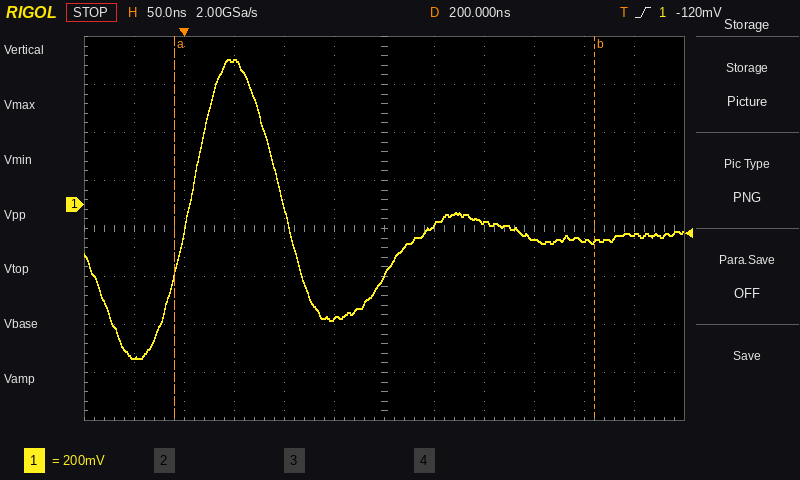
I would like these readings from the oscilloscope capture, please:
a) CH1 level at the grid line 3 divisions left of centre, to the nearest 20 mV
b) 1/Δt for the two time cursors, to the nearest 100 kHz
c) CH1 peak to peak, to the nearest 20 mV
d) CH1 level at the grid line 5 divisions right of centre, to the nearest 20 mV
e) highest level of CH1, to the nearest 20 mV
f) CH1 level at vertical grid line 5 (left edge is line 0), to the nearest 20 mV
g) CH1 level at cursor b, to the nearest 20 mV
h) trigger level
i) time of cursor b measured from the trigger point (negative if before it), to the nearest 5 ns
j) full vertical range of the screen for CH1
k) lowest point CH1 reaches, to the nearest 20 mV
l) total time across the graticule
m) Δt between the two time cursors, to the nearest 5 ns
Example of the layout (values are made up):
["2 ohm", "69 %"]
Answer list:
["600 mV", "2.4 MHz", "1.24 V", "-120 mV", "600 mV", "-480 mV", "-160 mV", "-120 mV", "+410 ns", "1.6 V", "-640 mV", "600 ns", "420 ns"]
